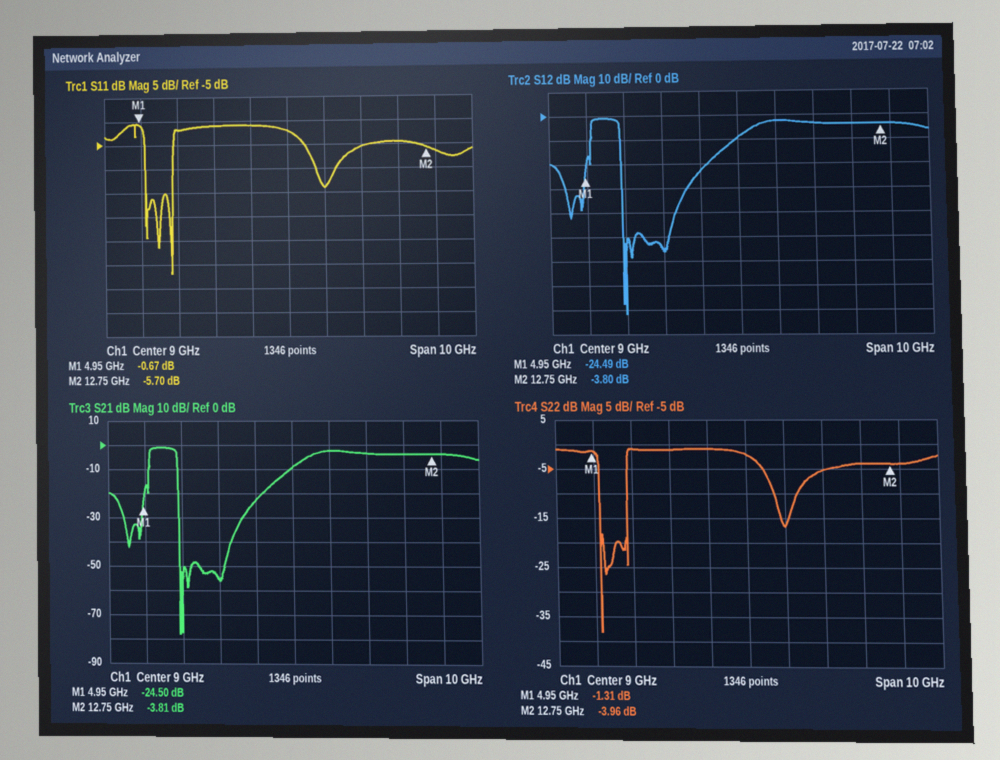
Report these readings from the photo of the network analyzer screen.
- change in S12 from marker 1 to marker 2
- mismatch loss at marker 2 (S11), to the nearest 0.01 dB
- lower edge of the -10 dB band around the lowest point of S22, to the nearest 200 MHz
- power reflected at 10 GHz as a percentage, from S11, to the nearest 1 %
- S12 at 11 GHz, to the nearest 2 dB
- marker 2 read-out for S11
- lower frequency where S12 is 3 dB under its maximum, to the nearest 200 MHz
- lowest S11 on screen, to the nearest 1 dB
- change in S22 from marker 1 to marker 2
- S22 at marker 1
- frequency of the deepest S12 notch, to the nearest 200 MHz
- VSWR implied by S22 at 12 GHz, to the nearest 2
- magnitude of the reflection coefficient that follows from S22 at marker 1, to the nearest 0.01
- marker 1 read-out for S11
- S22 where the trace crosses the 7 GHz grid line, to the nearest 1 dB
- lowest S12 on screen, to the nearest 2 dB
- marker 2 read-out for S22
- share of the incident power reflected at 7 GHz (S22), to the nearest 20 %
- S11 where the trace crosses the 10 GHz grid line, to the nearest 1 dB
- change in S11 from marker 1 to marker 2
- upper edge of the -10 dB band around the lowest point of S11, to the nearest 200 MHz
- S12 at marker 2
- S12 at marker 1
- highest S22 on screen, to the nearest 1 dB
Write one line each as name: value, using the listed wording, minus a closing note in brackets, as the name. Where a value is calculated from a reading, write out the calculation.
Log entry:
change in S12 from marker 1 to marker 2: -3.8 − (-24.49) = 20.69 dB
mismatch loss at marker 2 (S11), to the nearest 0.01 dB: −10 log10(1 − 10^(-5.7/10)) ≈ 1.36 dB
lower edge of the -10 dB band around the lowest point of S22, to the nearest 200 MHz: 5.2 GHz
power reflected at 10 GHz as a percentage, from S11, to the nearest 1 %: 10^(-14/10) ≈ 4 %
S12 at 11 GHz, to the nearest 2 dB: -4 dB
marker 2 read-out for S11: -5.70 dB
lower frequency where S12 is 3 dB under its maximum, to the nearest 200 MHz: 5.2 GHz
lowest S11 on screen, to the nearest 1 dB: -32 dB
change in S22 from marker 1 to marker 2: -3.96 − (-1.31) = -2.65 dB
S22 at marker 1: -1.31 dB
frequency of the deepest S12 notch, to the nearest 200 MHz: 6.0 GHz
VSWR implied by S22 at 12 GHz, to the nearest 2: |Γ| = 10^(-4/20) = 0.6310; VSWR = (1 + 0.6310)/(1 − 0.6310) ≈ 4
magnitude of the reflection coefficient that follows from S22 at marker 1, to the nearest 0.01: 10^(-1.31/20) ≈ 0.86
marker 1 read-out for S11: -0.67 dB
S22 where the trace crosses the 7 GHz grid line, to the nearest 1 dB: -1 dB
lowest S12 on screen, to the nearest 2 dB: -82 dB
marker 2 read-out for S22: -3.96 dB
share of the incident power reflected at 7 GHz (S22), to the nearest 20 %: 10^(-1/10) ≈ 79.4 %, so 80 % to the nearest 20 %
S11 where the trace crosses the 10 GHz grid line, to the nearest 1 dB: -14 dB
change in S11 from marker 1 to marker 2: -5.7 − (-0.67) = -5.03 dB
upper edge of the -10 dB band around the lowest point of S11, to the nearest 200 MHz: 5.8 GHz
S12 at marker 2: -3.80 dB
S12 at marker 1: -24.49 dB
highest S22 on screen, to the nearest 1 dB: -1 dB
